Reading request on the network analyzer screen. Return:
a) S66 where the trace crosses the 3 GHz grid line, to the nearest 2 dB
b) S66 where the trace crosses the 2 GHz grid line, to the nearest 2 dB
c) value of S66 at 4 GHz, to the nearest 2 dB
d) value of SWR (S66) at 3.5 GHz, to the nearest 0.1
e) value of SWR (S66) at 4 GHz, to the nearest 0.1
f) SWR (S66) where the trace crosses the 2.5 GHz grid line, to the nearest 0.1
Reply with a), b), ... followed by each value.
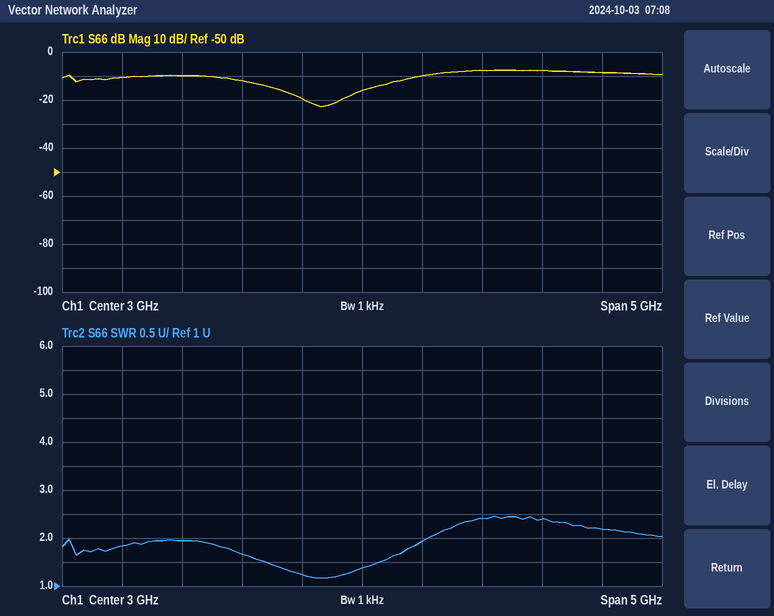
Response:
a) -16 dB
b) -12 dB
c) -8 dB
d) 1.9
e) 2.4
f) 1.2
